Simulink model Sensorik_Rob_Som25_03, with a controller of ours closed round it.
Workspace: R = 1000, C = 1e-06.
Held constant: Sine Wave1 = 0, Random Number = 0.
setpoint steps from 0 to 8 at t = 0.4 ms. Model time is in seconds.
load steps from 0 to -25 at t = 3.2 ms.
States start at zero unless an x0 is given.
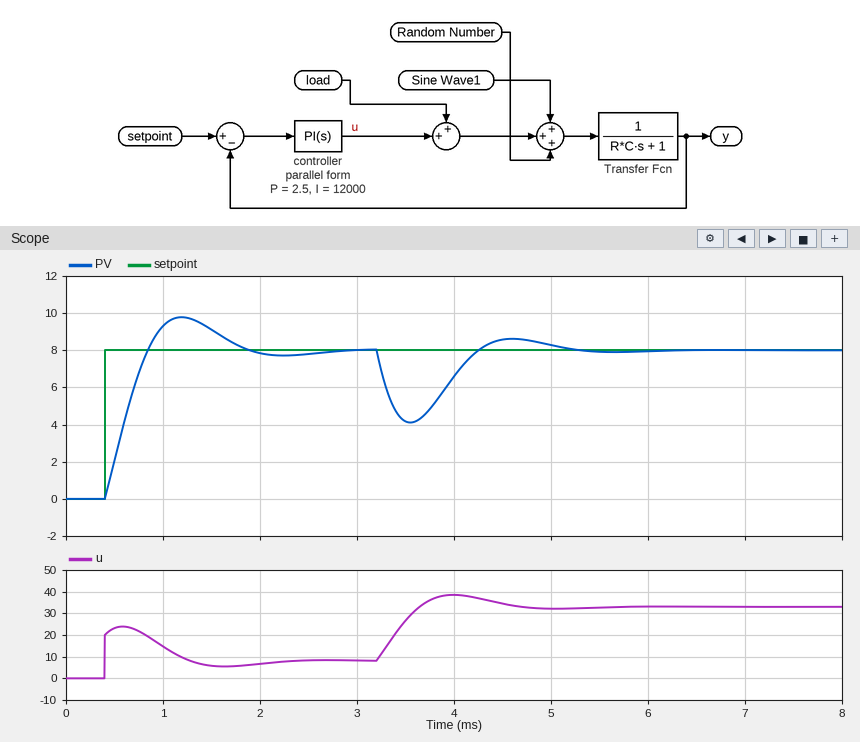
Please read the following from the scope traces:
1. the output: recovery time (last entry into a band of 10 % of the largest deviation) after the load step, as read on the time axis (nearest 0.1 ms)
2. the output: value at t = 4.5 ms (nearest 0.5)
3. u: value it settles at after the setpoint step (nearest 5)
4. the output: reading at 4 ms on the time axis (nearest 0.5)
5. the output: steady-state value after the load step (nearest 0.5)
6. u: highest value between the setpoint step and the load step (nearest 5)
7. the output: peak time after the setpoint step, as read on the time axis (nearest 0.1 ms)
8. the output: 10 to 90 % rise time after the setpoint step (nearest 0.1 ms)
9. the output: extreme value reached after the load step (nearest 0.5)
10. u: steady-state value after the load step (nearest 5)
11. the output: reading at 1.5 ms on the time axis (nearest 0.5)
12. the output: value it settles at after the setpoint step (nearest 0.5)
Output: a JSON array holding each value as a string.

["4.9 ms", "8.5", "10", "6.5", "8.0", "25", "1.2 ms", "0.3 ms", "4.0", "35", "9.0", "8.0"]
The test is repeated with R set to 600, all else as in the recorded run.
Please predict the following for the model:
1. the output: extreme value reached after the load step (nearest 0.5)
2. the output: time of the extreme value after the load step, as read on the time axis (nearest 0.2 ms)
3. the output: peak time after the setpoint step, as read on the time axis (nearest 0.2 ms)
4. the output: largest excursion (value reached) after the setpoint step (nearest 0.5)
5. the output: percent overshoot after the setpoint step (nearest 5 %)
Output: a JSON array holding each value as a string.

["3.5", "3.4 ms", "1.0 ms", "9.0", "15 %"]
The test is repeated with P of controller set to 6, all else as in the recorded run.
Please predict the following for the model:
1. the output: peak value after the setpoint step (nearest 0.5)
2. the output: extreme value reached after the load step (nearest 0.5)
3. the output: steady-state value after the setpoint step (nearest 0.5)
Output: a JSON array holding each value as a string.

["8.5", "5.5", "8.0"]
